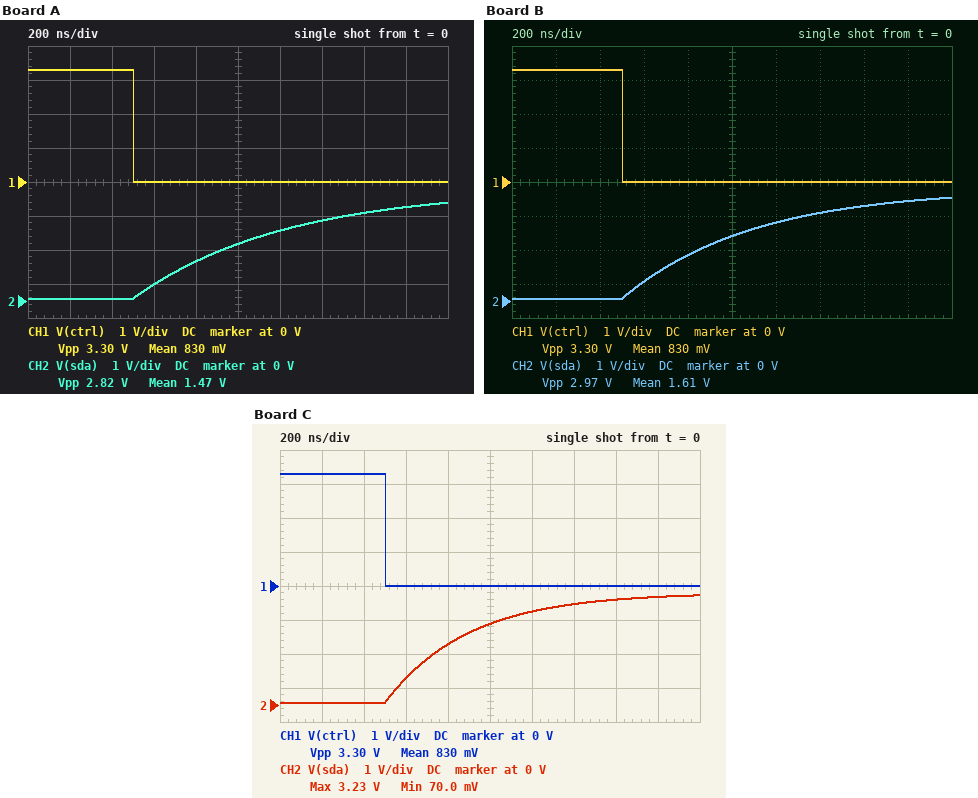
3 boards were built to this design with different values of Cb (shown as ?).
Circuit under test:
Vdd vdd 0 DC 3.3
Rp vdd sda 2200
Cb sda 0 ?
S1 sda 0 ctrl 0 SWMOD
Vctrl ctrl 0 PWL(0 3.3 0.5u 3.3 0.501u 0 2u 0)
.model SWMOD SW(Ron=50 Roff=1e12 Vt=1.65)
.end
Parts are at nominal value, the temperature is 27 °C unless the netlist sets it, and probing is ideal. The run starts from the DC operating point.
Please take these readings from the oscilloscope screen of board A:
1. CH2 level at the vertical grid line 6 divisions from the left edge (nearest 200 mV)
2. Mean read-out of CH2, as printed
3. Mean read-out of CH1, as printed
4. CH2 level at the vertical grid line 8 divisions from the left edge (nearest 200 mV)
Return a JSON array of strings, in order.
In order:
["2.0 V", "1.47 V", "830 mV", "2.6 V"]
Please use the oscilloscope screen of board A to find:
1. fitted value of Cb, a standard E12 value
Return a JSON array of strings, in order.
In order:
["330 pF"]
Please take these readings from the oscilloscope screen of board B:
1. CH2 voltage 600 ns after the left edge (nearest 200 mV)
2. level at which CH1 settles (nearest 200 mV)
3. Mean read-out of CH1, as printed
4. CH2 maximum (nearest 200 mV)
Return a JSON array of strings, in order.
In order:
["600 mV", "0 V", "830 mV", "3.0 V"]
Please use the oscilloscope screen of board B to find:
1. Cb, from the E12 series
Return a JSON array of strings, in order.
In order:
["270 pF"]
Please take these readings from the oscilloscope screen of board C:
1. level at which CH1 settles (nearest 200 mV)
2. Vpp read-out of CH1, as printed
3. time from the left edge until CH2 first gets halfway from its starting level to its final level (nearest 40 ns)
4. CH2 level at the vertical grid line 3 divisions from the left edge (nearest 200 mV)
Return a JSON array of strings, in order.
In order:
["0 V", "3.30 V", "760 ns", "800 mV"]
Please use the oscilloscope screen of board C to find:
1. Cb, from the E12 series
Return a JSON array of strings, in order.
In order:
["180 pF"]
